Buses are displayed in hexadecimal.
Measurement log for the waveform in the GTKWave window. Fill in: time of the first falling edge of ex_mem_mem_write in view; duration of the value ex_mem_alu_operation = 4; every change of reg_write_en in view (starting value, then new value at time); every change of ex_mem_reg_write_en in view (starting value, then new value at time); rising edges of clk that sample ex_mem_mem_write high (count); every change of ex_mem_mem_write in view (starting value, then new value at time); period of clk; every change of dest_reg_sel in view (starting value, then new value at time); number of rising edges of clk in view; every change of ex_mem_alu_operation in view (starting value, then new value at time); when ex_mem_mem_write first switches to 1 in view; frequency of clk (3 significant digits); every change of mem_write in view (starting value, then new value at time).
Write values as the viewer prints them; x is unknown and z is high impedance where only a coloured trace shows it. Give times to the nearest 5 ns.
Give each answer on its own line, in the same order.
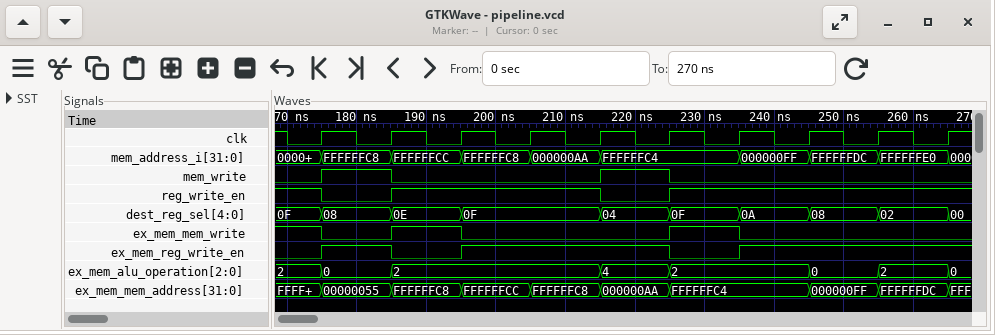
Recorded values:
175 ns
10 ns
1, 0 at 175 ns, 1 at 185 ns, 0 at 215 ns, 1 at 225 ns
0, 1 at 175 ns, 0 at 185 ns, 1 at 195 ns, 0 at 225 ns, 1 at 235 ns
3
1, 0 at 175 ns, 1 at 185 ns, 0 at 195 ns, 1 at 225 ns, 0 at 235 ns
10 ns
0F, 08 at 175 ns, 0E at 185 ns, 0F at 195 ns, 04 at 215 ns, 0F at 225 ns, 0A at 235 ns, 08 at 245 ns, 02 at 255 ns, 00 at 265 ns
10
2, 0 at 175 ns, 2 at 185 ns, 4 at 215 ns, 2 at 225 ns, 0 at 245 ns, 2 at 255 ns, 0 at 265 ns
185 ns
100 MHz
0, 1 at 175 ns, 0 at 185 ns, 1 at 215 ns, 0 at 225 ns
